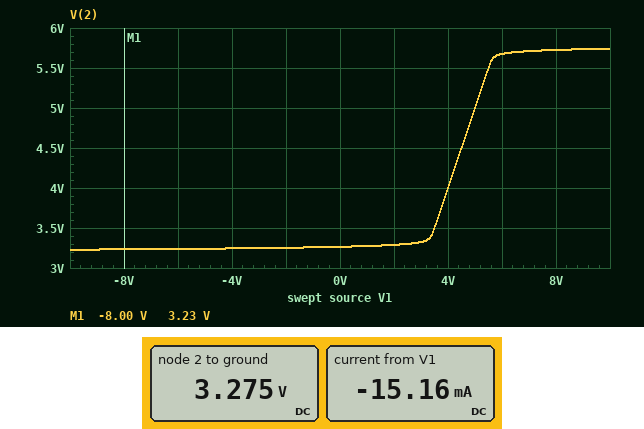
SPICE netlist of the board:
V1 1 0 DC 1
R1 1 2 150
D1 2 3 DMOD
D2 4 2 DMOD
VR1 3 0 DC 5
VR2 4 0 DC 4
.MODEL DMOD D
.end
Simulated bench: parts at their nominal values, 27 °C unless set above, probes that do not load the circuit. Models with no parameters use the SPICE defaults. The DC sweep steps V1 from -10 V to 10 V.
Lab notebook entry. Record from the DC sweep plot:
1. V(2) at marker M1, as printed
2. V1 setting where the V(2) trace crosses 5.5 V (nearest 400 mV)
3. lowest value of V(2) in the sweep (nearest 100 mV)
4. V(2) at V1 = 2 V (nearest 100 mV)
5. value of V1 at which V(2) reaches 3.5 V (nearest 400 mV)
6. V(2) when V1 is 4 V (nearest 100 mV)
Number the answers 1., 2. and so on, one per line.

1. 3.23 V
2. 5.6 V
3. 3.2 V
4. 3.3 V
5. 3.6 V
6. 4.0 V
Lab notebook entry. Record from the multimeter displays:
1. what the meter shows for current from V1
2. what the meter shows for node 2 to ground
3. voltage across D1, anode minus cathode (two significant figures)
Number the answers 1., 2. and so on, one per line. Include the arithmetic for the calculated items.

1. -15.16 mA
2. 3.275 V
3. 3.275 V - 5 V = -1.7 V
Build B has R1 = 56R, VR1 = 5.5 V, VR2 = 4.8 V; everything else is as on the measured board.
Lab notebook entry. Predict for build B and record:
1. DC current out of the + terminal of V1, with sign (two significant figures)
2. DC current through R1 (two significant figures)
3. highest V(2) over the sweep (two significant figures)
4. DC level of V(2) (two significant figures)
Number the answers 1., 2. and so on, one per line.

1. -54 mA
2. 54 mA
3. 6.3 V
4. 4.0 V
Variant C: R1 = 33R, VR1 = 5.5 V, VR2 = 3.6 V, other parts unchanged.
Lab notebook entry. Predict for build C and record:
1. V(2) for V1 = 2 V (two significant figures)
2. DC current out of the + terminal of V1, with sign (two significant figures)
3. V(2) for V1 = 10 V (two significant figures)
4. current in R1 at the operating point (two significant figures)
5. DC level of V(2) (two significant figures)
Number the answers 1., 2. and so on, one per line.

1. 2.9 V
2. -56 mA
3. 6.3 V
4. 56 mA
5. 2.8 V
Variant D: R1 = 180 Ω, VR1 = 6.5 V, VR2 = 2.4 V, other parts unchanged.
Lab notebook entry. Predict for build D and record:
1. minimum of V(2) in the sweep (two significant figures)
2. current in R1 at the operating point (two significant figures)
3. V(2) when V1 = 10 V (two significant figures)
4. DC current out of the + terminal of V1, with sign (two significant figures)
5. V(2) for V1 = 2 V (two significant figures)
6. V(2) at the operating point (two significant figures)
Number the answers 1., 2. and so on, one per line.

1. 1.6 V
2. 3.9 mA
3. 7.2 V
4. -3.9 mA
5. 2.0 V
6. 1.7 V
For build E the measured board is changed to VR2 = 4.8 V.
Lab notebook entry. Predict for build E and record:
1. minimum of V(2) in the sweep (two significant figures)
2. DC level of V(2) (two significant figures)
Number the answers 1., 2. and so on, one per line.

1. 4.0 V
2. 4.1 V
